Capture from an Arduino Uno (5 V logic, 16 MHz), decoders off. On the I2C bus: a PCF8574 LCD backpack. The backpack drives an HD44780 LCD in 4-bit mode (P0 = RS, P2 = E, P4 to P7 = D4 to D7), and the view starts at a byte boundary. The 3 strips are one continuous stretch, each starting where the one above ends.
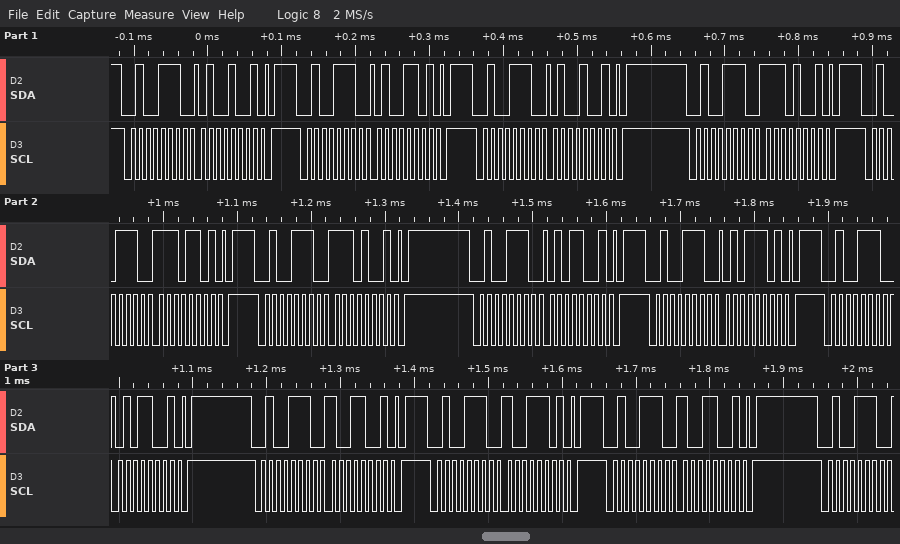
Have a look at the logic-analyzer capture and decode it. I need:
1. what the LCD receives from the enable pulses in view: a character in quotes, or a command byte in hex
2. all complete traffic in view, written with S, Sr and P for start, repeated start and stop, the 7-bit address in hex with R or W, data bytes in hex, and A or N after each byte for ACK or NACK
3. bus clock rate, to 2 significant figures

'N' 'Y'
S 27W A 49 A P S 27W A 4D A P S 27W A 49 A P S 27W A E9 A P S 27W A ED A P S 27W A E9 A P S 27W A 59 A P S 27W A 5D A P S 27W A 59 A P S 27W A 99 A P S 27W A 9D A P S 27W A 99 A P S 27W A
100 kHz
